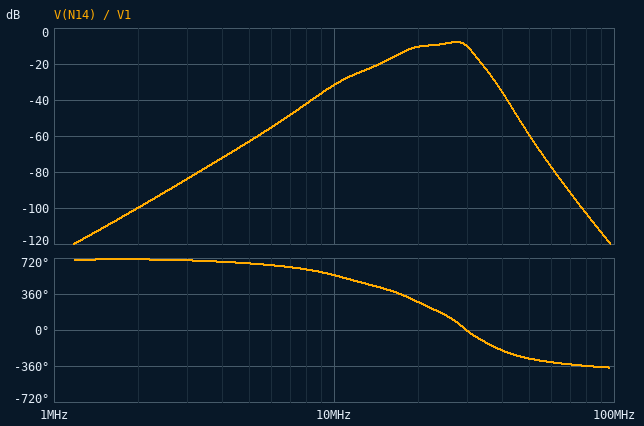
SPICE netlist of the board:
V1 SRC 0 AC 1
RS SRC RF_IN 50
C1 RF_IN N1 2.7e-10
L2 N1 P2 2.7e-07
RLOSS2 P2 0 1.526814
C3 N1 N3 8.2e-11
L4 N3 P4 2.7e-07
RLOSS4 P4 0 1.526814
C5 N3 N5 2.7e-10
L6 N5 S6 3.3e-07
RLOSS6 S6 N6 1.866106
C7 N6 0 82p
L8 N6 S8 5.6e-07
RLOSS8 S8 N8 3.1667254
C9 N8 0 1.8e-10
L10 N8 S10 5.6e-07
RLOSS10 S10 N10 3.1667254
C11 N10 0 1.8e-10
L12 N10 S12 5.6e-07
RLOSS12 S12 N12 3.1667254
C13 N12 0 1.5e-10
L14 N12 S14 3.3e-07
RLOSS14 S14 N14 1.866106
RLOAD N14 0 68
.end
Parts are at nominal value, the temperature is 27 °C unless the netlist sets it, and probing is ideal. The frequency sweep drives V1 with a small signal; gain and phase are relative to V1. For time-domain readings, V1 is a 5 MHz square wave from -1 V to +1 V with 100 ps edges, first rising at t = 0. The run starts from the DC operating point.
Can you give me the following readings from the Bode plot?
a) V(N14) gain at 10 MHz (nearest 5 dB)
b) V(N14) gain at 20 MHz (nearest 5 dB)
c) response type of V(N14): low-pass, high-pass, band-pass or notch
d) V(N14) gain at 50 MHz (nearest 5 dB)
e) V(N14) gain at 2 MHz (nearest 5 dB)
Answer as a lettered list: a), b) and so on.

a) -30 dB
b) -10 dB
c) band-pass
d) -60 dB
e) -100 dB
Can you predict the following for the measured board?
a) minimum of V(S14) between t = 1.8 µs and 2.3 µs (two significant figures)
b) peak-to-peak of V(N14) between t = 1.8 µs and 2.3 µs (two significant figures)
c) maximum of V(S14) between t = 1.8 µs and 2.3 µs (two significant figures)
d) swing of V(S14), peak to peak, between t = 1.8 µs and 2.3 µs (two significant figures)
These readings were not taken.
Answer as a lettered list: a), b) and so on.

a) -160 mV
b) 310 mV
c) 160 mV
d) 320 mV
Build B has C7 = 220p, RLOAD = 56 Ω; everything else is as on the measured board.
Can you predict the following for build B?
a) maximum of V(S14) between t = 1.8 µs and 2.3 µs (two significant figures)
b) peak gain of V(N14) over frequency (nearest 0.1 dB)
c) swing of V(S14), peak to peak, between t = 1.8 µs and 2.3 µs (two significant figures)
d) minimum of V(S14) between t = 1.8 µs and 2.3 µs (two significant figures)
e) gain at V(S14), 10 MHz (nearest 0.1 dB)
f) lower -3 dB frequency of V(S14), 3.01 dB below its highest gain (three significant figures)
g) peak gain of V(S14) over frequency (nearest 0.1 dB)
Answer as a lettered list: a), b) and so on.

a) 140 mV
b) -9.4 dB
c) 290 mV
d) -140 mV
e) -33.8 dB
f) 17.0 MHz
g) -9.1 dB
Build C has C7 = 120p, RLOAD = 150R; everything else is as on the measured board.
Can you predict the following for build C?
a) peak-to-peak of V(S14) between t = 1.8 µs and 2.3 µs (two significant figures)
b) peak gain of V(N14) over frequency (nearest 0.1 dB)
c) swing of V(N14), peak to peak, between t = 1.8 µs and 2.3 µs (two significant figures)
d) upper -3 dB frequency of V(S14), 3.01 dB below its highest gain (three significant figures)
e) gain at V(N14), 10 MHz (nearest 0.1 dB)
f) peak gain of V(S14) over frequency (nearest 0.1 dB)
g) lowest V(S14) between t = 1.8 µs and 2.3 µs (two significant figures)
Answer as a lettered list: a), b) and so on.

a) 440 mV
b) -4.0 dB
c) 430 mV
d) 30.0 MHz
e) -27.5 dB
f) -3.9 dB
g) -220 mV
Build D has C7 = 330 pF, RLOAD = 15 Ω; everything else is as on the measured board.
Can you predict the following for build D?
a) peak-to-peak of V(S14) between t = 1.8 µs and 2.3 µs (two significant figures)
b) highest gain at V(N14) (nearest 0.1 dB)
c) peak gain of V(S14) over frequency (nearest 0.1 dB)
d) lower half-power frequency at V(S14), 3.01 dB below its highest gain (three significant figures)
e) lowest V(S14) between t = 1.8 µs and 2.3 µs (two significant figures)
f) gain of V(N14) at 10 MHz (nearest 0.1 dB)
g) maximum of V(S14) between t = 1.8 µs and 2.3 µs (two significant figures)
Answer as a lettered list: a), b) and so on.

a) 130 mV
b) -16.7 dB
c) -15.7 dB
d) 16.7 MHz
e) -64 mV
f) -45.0 dB
g) 64 mV
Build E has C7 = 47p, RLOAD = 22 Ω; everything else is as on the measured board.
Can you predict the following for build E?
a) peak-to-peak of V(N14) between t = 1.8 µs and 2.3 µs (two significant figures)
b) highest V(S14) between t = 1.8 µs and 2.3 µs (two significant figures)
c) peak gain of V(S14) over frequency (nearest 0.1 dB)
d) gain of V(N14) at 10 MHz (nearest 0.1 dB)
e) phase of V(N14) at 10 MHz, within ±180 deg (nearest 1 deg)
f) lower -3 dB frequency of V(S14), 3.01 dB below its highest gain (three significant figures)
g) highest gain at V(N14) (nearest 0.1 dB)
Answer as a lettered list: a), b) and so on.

a) 150 mV
b) 82 mV
c) -12.6 dB
d) -39.8 dB
e) -161 deg
f) 20.9 MHz
g) -13.3 dB
